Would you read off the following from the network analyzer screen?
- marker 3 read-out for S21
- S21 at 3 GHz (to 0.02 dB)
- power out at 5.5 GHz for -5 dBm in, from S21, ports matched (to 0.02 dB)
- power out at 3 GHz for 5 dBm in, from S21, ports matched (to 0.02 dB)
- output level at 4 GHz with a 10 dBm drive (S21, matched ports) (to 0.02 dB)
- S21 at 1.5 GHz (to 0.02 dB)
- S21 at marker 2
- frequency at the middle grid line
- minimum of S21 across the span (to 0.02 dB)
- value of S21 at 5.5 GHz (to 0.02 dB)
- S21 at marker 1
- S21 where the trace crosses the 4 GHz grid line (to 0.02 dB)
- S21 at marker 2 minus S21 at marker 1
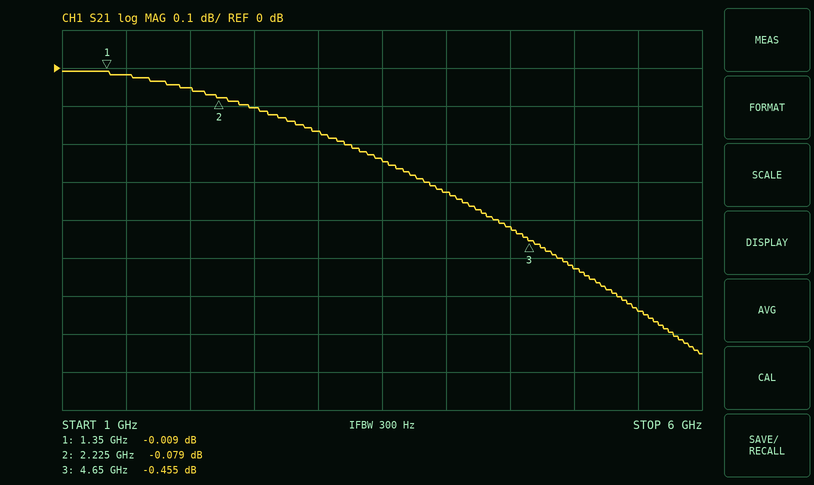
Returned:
-0.455 dB
-0.16 dB
-5.64 dBm
4.84 dBm
9.68 dBm
-0.02 dB
-0.079 dB
3.5 GHz
-0.76 dB
-0.64 dB
-0.009 dB
-0.32 dB
-0.070 dB
